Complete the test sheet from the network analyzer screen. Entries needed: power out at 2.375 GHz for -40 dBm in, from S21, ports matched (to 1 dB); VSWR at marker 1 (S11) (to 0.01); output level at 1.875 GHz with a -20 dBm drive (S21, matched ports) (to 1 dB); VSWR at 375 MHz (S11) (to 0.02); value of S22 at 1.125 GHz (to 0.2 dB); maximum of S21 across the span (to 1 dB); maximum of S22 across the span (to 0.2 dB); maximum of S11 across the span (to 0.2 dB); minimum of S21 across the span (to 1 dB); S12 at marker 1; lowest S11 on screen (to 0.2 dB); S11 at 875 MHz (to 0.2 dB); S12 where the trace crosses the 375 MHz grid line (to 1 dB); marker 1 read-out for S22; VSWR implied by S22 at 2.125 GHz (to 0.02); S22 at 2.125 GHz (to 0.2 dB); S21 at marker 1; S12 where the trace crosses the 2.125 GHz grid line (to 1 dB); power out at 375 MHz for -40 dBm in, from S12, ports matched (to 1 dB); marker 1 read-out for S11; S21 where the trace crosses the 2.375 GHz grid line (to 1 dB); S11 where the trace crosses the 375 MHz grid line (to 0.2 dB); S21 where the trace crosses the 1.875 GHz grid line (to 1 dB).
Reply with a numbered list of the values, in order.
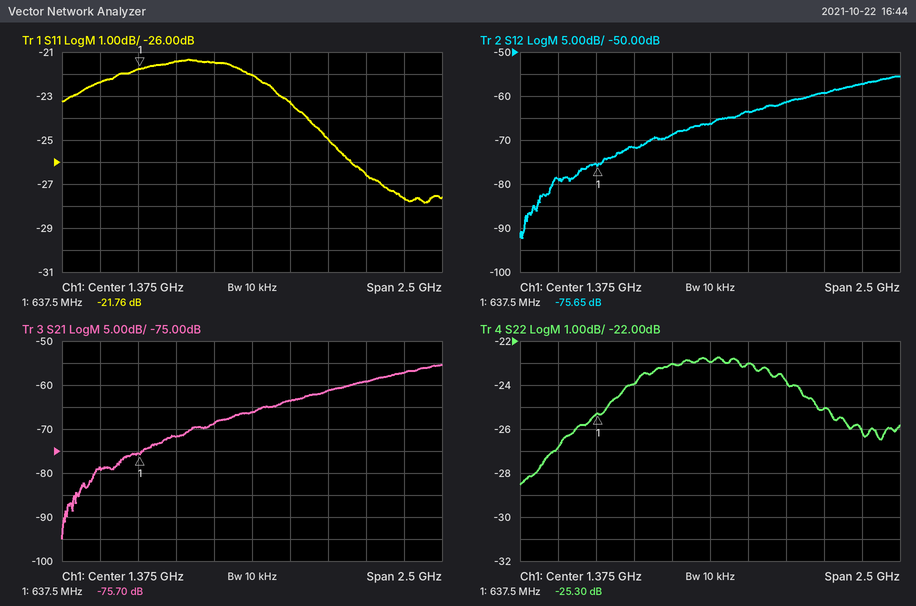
1. -97 dBm
2. 1.18
3. -81 dBm
4. 1.16
5. -23.0 dB
6. -55 dB
7. -22.8 dB
8. -21.4 dB
9. -95 dB
10. -75.65 dB
11. -27.8 dB
12. -21.4 dB
13. -79 dB
14. -25.30 dB
15. 1.12
16. -25.0 dB
17. -75.70 dB
18. -59 dB
19. -119 dBm
20. -21.76 dB
21. -57 dB
22. -22.4 dB
23. -61 dB
